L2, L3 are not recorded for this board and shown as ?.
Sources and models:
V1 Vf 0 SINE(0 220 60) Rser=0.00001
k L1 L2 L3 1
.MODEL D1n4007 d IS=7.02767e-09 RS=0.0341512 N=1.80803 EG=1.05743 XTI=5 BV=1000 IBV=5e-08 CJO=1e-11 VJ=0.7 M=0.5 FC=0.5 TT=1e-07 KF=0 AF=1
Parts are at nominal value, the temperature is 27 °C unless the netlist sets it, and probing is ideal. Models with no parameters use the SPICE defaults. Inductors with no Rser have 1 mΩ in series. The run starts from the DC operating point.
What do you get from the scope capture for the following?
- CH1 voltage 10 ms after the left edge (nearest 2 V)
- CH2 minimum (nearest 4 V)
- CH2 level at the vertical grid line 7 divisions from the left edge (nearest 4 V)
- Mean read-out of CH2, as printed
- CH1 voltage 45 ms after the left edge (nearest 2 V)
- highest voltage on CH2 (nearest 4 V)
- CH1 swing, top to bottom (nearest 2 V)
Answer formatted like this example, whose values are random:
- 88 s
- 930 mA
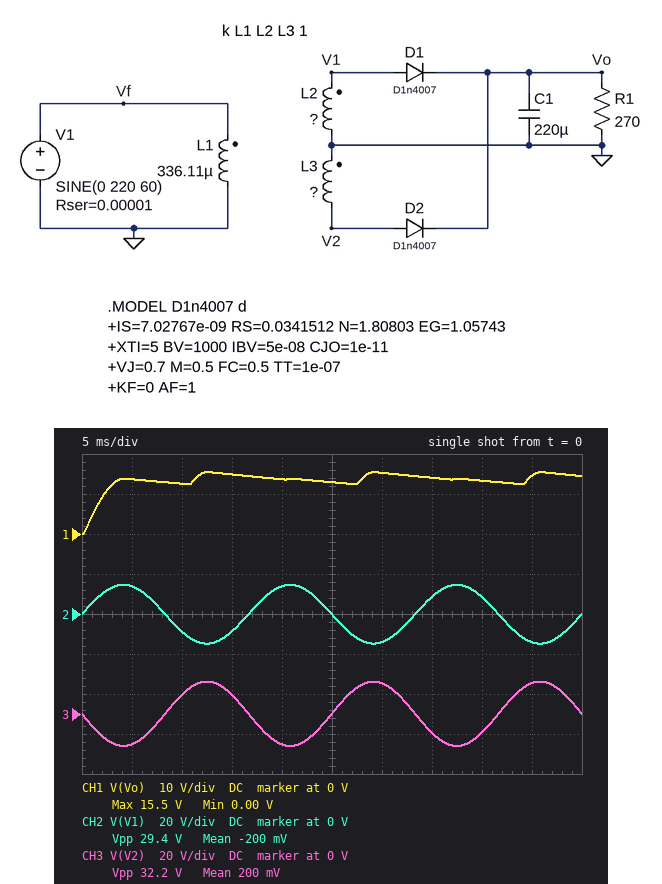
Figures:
- 12 V
- -16 V
- 8 V
- -200 mV
- 14 V
- 16 V
- 16 V
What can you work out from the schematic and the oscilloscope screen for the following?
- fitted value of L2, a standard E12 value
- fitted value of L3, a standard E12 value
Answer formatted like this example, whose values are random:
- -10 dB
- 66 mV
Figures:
- 1.5 µH
- 1.8 µH
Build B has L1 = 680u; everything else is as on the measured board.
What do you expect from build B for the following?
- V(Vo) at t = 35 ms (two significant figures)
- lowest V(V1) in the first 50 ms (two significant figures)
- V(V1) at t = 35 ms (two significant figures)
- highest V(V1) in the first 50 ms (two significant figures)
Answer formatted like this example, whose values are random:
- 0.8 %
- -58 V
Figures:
- 9.7 V
- -10 V
- 6.1 V
- 10 V
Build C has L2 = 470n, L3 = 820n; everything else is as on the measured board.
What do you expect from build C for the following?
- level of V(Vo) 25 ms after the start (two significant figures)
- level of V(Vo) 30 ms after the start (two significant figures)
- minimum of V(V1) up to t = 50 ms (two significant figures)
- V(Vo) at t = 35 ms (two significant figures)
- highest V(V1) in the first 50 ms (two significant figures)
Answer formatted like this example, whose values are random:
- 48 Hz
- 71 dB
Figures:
- 8.3 V
- 10 V
- -8.3 V
- 9.3 V
- 8.2 V
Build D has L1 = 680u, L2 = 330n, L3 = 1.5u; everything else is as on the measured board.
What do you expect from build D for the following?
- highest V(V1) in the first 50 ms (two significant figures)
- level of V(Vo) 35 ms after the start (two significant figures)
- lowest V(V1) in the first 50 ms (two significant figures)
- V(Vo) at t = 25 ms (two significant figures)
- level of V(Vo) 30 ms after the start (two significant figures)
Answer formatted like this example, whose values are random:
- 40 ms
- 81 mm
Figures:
- 4.8 V
- 8.8 V
- -4.9 V
- 7.8 V
- 9.5 V
